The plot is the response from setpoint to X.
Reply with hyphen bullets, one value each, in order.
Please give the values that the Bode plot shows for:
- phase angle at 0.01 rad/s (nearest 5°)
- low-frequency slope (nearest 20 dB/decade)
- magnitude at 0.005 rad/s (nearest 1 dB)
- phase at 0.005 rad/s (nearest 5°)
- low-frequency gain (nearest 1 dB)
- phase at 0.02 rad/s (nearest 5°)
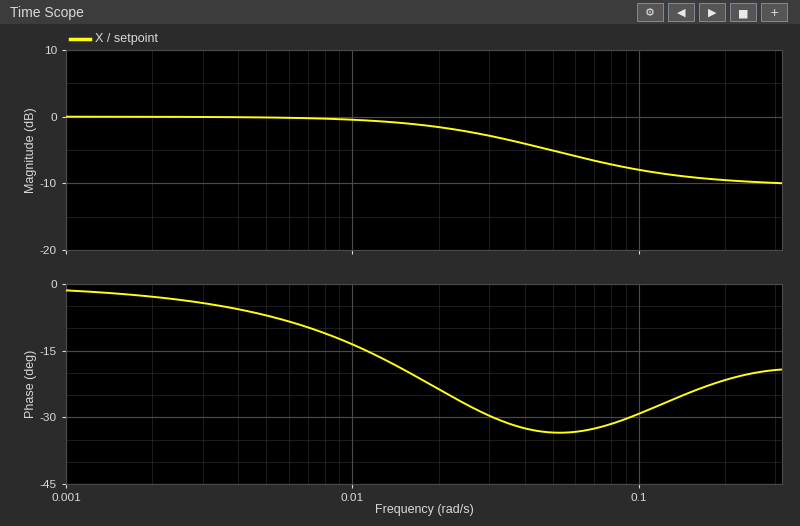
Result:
- -15°
- 0 dB/decade
- 0 dB
- -5°
- 0 dB
- -25°
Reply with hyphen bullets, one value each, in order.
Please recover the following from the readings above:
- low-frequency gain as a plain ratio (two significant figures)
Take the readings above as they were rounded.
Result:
- 1.0
